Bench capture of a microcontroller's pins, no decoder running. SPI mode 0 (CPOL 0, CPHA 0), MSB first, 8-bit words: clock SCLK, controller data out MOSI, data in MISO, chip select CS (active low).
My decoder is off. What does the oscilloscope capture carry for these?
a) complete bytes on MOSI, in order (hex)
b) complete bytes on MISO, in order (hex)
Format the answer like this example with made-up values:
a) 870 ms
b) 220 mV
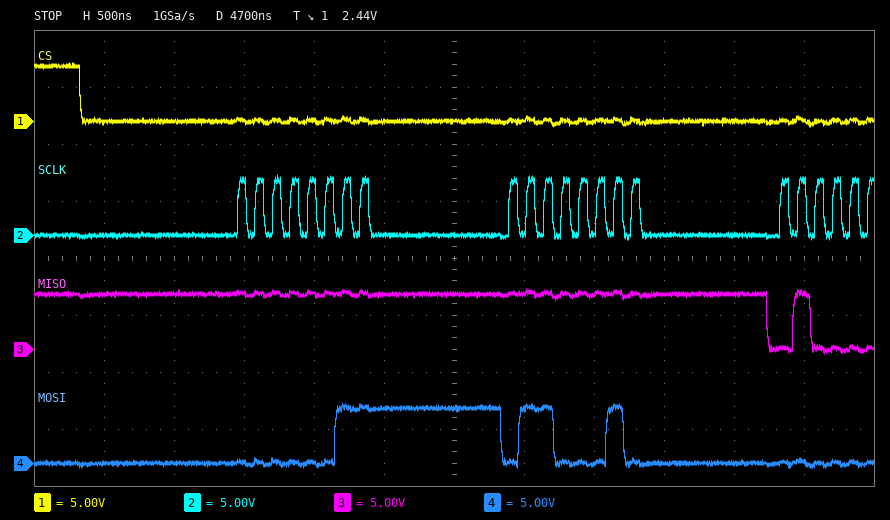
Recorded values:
a) 03 62
b) FF FF
